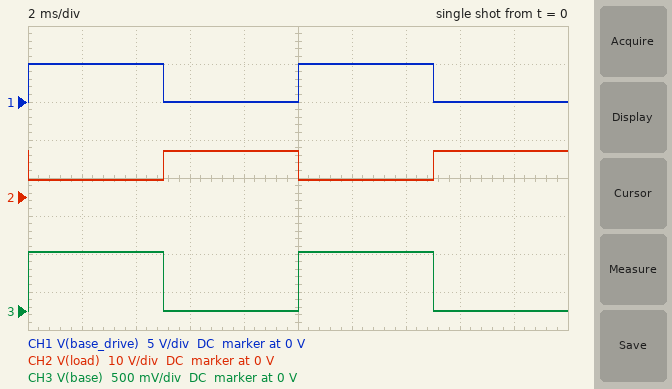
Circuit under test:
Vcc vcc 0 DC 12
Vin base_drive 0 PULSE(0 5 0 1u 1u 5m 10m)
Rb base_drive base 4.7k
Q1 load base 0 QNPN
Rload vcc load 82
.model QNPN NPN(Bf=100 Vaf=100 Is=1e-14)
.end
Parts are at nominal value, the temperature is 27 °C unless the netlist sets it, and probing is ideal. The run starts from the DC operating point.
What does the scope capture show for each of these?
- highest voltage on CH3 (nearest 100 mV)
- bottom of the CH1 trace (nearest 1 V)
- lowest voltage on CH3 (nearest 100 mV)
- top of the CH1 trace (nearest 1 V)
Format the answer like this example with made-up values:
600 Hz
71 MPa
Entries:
800 mV
0 V
0 V
5 V
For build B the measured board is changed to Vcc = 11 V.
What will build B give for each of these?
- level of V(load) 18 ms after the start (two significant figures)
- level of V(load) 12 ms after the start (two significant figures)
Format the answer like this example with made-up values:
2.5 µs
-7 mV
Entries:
11 V
3.4 V
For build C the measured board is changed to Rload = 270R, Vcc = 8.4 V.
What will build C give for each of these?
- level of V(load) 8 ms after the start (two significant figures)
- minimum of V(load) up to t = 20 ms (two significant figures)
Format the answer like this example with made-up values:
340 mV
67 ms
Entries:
8.4 V
100 mV
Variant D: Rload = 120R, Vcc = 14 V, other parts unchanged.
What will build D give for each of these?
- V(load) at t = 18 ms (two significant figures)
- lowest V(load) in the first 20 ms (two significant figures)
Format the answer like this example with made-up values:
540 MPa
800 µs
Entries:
14 V
3.0 V
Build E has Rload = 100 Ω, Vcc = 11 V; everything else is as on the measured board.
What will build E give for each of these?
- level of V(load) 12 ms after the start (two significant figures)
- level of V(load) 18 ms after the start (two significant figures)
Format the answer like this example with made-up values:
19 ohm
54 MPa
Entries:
1.9 V
11 V
